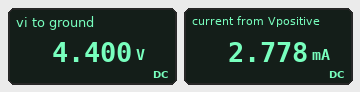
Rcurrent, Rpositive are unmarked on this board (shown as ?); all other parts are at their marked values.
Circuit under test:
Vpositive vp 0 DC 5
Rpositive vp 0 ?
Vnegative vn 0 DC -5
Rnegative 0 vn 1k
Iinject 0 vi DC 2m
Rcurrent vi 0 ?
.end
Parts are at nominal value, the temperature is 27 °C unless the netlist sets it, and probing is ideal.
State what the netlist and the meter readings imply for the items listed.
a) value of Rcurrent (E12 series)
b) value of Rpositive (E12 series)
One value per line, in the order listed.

2.2 kΩ
1.8 kΩ
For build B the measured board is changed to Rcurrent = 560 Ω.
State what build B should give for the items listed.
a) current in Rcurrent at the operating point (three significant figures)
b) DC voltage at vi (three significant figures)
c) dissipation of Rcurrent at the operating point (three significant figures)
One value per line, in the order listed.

2.00 mA
1.12 V
2.24 mW
